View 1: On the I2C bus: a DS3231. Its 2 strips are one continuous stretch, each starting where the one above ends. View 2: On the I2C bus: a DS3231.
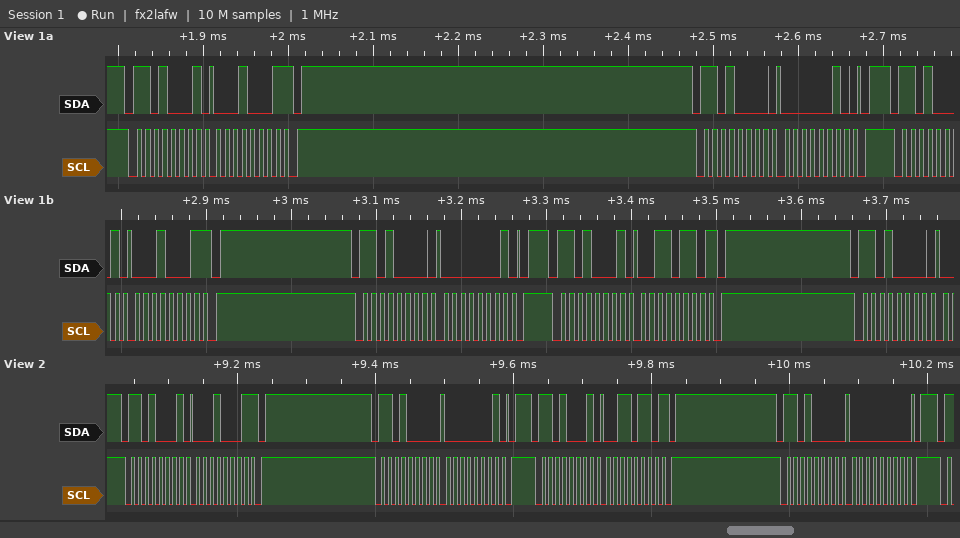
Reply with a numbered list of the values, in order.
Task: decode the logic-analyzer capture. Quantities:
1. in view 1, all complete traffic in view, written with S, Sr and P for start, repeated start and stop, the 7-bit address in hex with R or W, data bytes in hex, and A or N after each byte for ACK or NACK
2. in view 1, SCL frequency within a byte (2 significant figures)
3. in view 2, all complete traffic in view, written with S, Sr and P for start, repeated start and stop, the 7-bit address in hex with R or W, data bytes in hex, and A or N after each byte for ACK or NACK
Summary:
1. S 68R A 11 N P S 68W A 02 A P S 68R A 11 N P S 68W A 01 A P S 68R A 36 N P S 68W A
2. 100 kHz
3. S 68R A 11 N P S 68W A 01 A P S 68R A 36 N P S 68W A 00 A P
